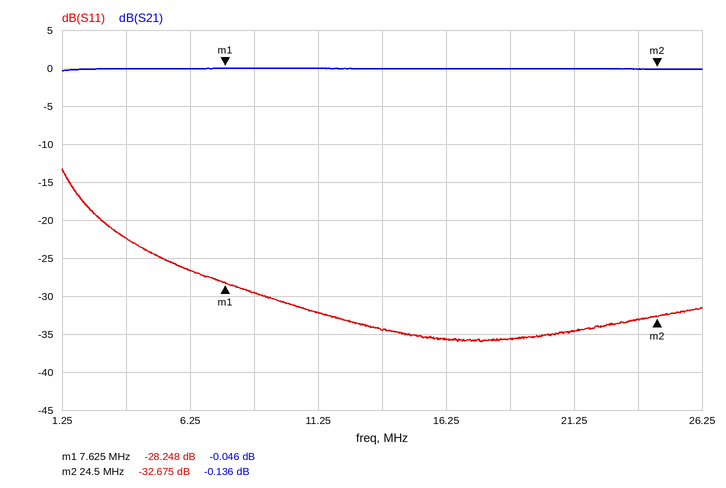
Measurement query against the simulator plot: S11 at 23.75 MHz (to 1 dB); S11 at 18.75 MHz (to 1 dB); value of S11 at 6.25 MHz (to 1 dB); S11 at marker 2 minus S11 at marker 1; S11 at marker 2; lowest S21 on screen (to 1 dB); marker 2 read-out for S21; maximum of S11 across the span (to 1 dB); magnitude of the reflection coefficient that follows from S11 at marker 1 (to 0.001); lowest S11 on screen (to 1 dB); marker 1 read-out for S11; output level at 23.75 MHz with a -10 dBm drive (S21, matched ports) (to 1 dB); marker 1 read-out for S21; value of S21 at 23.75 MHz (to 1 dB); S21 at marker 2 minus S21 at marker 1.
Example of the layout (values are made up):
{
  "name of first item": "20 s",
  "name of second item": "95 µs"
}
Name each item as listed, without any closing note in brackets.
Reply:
{
  "S11 at 23.75 MHz": "-33 dB",
  "S11 at 18.75 MHz": "-36 dB",
  "value of S11 at 6.25 MHz": "-27 dB",
  "S11 at marker 2 minus S11 at marker 1": "-4.427 dB",
  "S11 at marker 2": "-32.675 dB",
  "lowest S21 on screen": "0 dB",
  "marker 2 read-out for S21": "-0.136 dB",
  "maximum of S11 across the span": "-13 dB",
  "magnitude of the reflection coefficient that follows from S11 at marker 1": "0.039",
  "lowest S11 on screen": "-36 dB",
  "marker 1 read-out for S11": "-28.248 dB",
  "output level at 23.75 MHz with a -10 dBm drive (S21, matched ports)": "-10 dBm",
  "marker 1 read-out for S21": "-0.046 dB",
  "value of S21 at 23.75 MHz": "0 dB",
  "S21 at marker 2 minus S21 at marker 1": "-0.090 dB"
}
